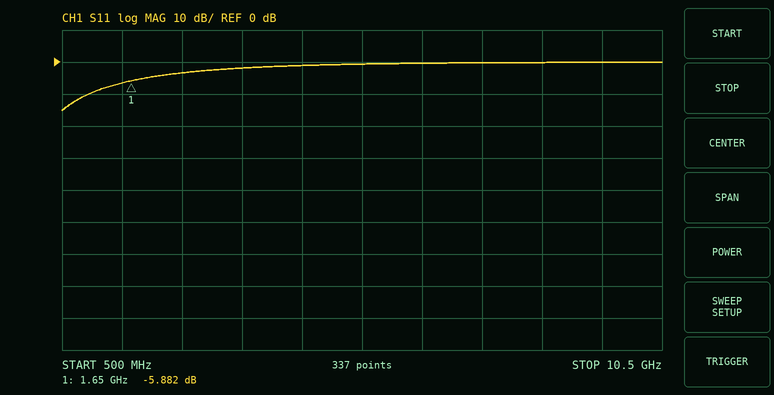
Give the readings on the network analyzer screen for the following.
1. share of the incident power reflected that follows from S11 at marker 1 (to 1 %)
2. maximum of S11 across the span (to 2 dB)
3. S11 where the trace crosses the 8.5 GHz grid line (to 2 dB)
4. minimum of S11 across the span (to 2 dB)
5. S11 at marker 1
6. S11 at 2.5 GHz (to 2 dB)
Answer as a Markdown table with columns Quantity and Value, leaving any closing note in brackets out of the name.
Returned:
| Quantity | Value |
|---|---|
| share of the incident power reflected that follows from S11 at marker 1 | 26 % |
| maximum of S11 across the span | 0 dB |
| S11 where the trace crosses the 8.5 GHz grid line | 0 dB |
| minimum of S11 across the span | -16 dB |
| S11 at marker 1 | -5.882 dB |
| S11 at 2.5 GHz | -4 dB |
